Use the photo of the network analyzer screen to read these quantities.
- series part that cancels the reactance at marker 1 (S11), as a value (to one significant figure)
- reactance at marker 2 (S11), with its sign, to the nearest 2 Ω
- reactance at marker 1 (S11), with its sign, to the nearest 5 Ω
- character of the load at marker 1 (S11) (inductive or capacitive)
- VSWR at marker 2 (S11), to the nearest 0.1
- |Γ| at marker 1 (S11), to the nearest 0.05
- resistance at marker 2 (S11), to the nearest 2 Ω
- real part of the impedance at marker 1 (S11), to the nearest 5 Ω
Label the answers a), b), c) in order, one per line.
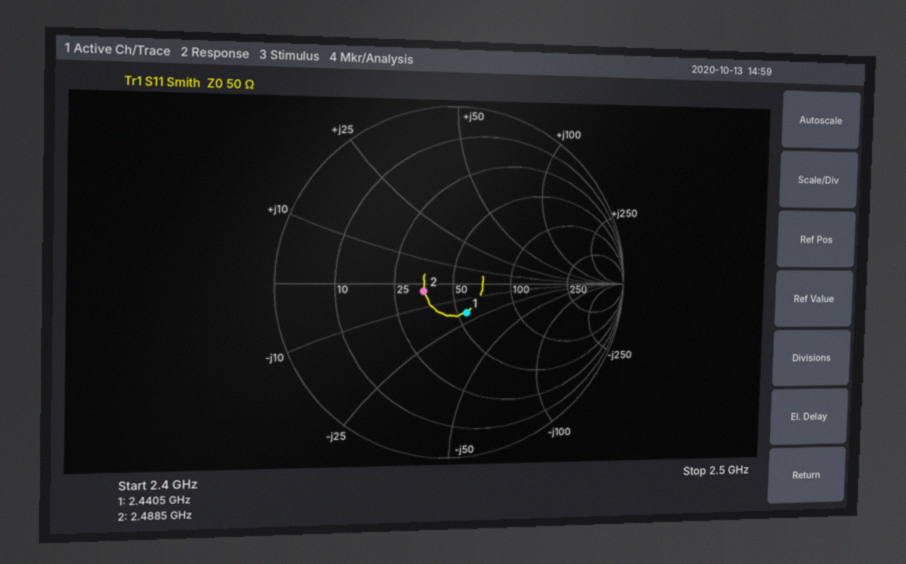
a) 1 nH
b) -4 Ω
c) -20 Ω
d) capacitive
e) 1.4
f) 0.20
g) 36 Ω
h) 55 Ω
